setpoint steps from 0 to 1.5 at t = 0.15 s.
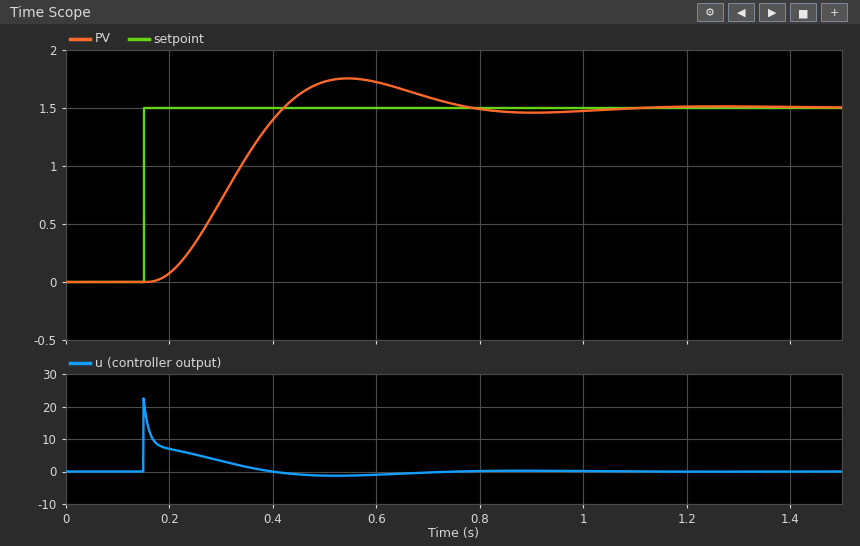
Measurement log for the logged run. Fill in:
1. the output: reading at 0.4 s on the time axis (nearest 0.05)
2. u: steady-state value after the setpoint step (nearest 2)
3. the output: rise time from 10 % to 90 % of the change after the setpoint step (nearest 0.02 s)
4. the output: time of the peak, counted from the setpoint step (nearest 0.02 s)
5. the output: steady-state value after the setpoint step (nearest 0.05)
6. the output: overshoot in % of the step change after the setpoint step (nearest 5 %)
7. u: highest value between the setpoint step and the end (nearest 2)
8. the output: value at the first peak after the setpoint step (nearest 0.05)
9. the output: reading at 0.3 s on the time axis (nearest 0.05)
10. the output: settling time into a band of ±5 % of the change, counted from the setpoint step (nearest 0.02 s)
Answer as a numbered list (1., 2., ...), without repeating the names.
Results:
1. 1.40
2. 0
3. 0.18 s
4. 0.40 s
5. 1.50
6. 15 %
7. 22
8. 1.75
9. 0.70
10. 0.56 s
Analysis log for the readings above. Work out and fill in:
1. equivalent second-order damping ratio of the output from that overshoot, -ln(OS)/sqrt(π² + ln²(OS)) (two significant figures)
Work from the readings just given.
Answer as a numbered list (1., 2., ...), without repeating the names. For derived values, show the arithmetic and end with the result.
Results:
1. ln(0.15) = -1.897; 1.897 / sqrt(9.870 + 3.599) = 0.52
